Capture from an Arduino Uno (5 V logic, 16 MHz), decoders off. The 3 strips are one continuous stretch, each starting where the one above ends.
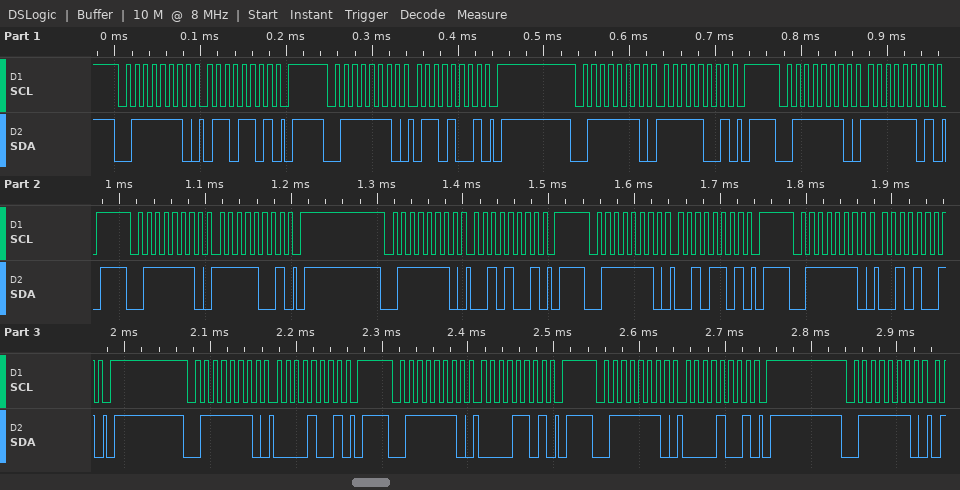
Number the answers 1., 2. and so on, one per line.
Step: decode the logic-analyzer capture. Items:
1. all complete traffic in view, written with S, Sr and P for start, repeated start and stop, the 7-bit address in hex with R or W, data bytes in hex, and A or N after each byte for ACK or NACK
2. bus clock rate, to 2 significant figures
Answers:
1. S 3FW A 6D A P S 3FW A 69 A P S 3FW A F9 A P S 3FW A FD A P S 3FW A F9 A P S 3FW A 29 A P S 3FW A 2D A P S 3FW A 29 A P S 3FW A 09 A P S 3FW A 0D A P S 3FW A 09 A P S 3FW A
2. 100 kHz
